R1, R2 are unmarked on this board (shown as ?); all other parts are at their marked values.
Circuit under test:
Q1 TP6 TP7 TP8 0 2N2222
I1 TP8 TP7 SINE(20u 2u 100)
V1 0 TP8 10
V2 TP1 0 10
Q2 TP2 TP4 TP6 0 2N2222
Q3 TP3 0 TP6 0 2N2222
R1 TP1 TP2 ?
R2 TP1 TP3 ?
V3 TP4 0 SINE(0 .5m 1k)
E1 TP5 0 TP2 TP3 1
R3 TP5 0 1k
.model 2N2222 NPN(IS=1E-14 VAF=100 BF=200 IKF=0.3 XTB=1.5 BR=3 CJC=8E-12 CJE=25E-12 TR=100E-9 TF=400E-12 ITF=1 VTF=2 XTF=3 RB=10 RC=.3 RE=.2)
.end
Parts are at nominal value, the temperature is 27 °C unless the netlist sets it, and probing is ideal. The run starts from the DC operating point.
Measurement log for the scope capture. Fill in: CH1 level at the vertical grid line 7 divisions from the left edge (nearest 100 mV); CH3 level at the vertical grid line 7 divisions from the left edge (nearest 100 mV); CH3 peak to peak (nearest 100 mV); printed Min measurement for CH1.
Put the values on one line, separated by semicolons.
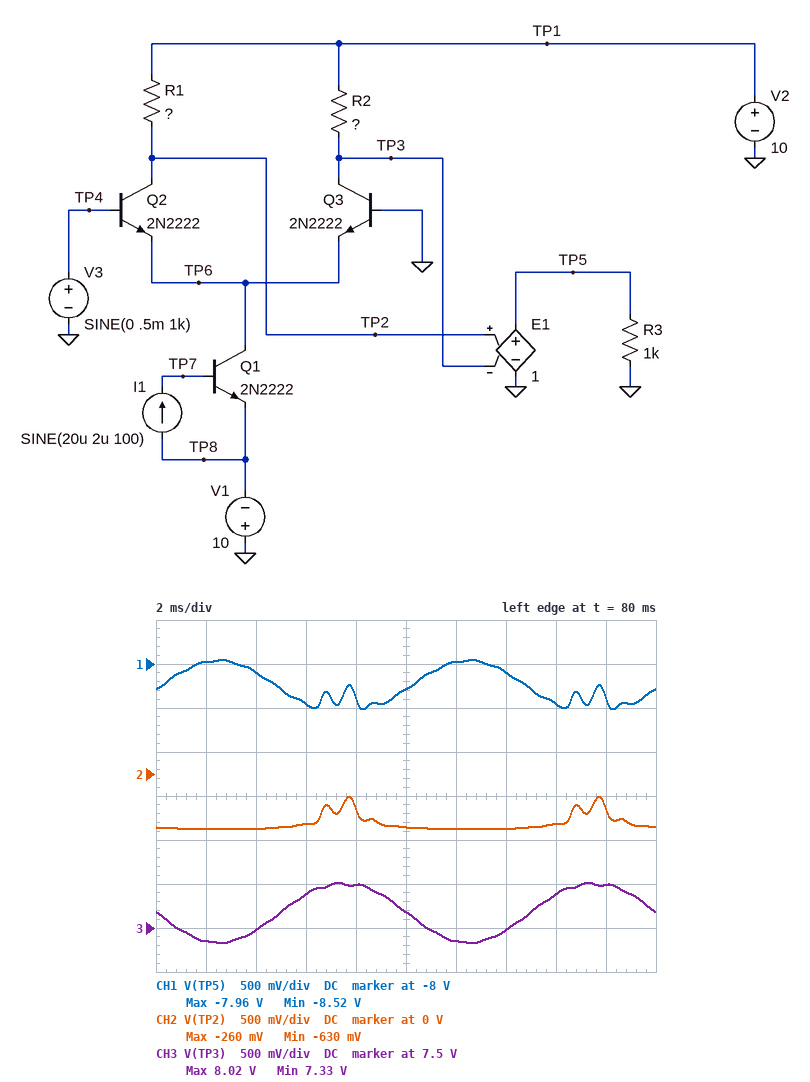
-8.1 V; 7.5 V; 700 mV; -8.52 V
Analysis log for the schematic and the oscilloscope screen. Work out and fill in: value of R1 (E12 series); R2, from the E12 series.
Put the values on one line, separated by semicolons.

5.6 kΩ; 1 kΩ
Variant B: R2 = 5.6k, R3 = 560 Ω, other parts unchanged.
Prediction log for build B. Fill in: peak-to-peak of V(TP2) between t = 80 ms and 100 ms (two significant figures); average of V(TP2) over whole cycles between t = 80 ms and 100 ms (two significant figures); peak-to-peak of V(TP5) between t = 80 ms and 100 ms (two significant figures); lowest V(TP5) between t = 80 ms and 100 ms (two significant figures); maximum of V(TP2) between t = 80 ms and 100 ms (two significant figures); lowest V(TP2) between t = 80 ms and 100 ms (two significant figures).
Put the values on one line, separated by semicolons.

74 mV; -640 mV; 12 mV; -5.8 mV; -590 mV; -670 mV
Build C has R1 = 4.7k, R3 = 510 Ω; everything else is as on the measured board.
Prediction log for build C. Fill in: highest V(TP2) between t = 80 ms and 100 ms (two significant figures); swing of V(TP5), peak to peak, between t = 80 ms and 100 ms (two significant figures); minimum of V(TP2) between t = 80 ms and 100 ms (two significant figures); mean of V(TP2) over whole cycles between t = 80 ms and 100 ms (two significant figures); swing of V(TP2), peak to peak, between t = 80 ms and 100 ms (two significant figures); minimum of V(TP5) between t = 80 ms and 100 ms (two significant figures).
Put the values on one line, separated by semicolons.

1.3 V; 1.5 V; -560 mV; 330 mV; 1.9 V; -8.1 V
